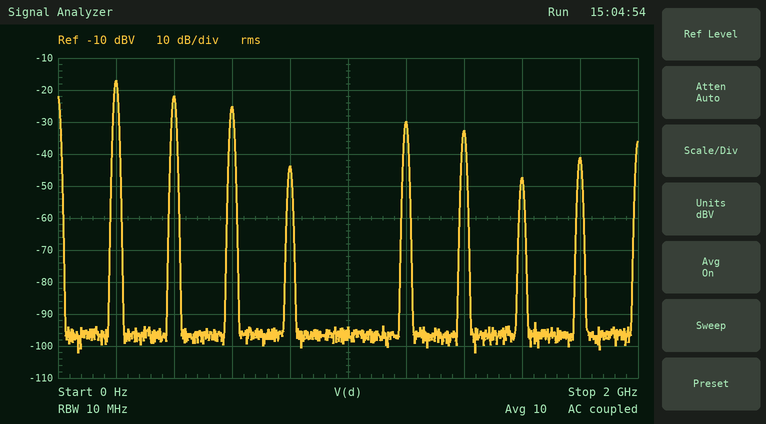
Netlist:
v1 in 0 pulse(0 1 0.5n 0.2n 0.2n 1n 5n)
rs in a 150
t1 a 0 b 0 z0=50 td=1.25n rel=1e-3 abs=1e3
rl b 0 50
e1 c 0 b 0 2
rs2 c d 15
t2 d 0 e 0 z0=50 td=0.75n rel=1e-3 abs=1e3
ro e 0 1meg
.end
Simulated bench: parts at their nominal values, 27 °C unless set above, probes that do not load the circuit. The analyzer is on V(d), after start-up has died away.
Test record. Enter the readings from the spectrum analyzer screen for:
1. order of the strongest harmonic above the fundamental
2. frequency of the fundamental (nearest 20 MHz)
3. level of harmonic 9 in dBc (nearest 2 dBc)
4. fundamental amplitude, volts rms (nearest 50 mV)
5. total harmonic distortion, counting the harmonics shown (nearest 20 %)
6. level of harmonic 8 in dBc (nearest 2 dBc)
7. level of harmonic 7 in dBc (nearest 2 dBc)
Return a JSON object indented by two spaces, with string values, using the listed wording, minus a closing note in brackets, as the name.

{
  "order of the strongest harmonic above the fundamental": "2",
  "frequency of the fundamental": "200 MHz",
  "level of harmonic 9 in dBc": "-24 dBc",
  "fundamental amplitude, volts rms": "150 mV",
  "total harmonic distortion, counting the harmonics shown": "80 %",
  "level of harmonic 8 in dBc": "-30 dBc",
  "level of harmonic 7 in dBc": "-16 dBc"
}
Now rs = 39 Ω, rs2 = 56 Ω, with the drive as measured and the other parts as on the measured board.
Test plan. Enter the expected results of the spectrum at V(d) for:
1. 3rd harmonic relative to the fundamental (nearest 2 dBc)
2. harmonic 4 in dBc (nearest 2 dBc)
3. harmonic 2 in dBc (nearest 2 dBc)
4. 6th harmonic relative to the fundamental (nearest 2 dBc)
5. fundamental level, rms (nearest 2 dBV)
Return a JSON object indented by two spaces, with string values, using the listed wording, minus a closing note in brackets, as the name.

{
  "3rd harmonic relative to the fundamental": "-4 dBc",
  "harmonic 4 in dBc": "-24 dBc",
  "harmonic 2 in dBc": "-8 dBc",
  "6th harmonic relative to the fundamental": "-10 dBc",
  "fundamental level, rms": "-14 dBV"
}
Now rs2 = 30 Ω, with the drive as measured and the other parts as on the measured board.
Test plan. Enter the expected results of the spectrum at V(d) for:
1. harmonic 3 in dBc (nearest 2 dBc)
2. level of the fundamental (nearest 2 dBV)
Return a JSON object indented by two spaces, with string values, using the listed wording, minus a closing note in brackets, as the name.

{
  "harmonic 3 in dBc": "-6 dBc",
  "level of the fundamental": "-18 dBV"
}
